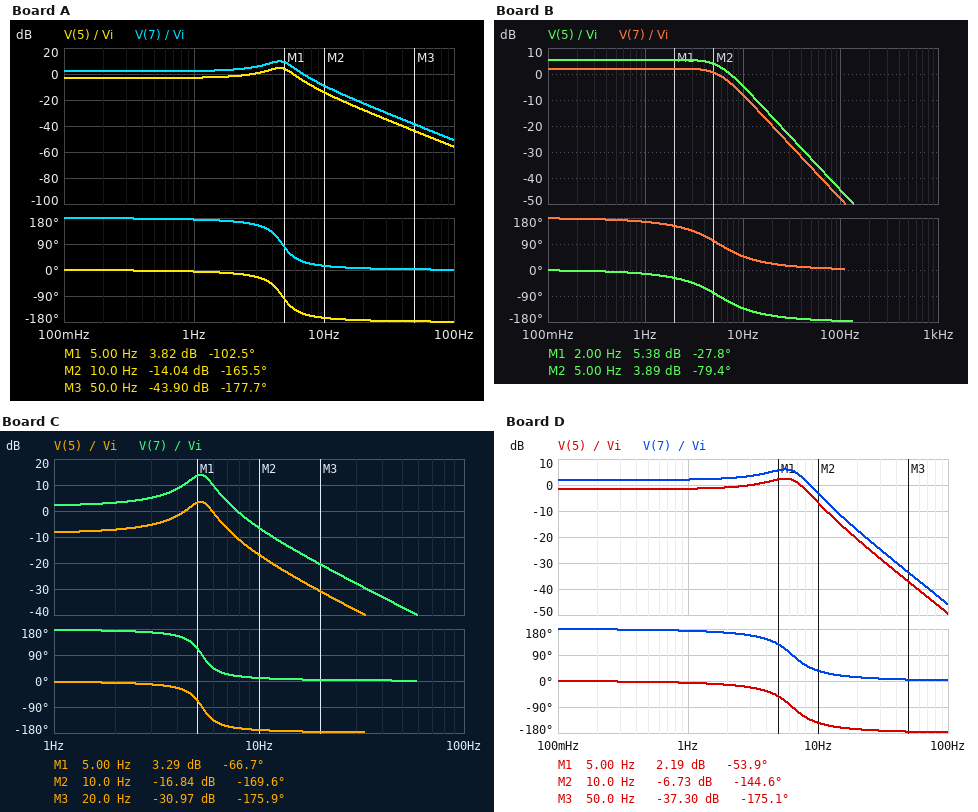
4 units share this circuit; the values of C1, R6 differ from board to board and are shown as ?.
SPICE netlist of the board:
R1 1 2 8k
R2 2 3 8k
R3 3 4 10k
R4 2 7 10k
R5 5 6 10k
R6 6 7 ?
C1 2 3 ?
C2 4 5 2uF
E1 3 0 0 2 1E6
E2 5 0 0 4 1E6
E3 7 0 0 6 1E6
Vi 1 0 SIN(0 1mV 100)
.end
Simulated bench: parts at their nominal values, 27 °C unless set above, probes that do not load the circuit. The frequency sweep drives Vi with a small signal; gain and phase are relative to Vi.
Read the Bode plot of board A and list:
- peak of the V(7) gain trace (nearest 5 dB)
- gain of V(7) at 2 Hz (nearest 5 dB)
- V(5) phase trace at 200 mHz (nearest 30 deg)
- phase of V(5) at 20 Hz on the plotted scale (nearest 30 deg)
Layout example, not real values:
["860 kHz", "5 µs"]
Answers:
["10 dB", "5 dB", "0 deg", "-180 deg"]
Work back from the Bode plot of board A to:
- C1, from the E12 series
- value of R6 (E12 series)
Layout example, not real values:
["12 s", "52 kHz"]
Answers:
["10 µF", "18 kΩ"]
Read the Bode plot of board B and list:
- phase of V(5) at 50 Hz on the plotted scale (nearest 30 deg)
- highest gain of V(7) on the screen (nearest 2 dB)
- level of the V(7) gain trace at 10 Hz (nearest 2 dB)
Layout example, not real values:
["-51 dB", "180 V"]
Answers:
["-180 deg", "2 dB", "-8 dB"]
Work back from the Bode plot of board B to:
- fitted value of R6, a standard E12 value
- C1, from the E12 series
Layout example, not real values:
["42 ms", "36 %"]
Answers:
["6.8 kΩ", "2.7 µF"]
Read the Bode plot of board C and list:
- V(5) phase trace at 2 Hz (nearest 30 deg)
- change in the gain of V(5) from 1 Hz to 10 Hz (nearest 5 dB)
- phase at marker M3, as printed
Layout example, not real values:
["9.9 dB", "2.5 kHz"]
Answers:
["0 deg", "-10 dB", "-175.9 deg"]
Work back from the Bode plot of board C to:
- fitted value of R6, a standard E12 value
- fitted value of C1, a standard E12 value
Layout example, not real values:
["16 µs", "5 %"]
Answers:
["33 kΩ", "15 µF"]
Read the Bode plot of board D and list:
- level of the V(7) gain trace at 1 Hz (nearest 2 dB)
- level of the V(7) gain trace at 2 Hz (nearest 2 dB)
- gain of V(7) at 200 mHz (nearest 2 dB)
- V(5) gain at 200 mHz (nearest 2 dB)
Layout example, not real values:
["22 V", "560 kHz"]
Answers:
["2 dB", "2 dB", "2 dB", "-2 dB"]
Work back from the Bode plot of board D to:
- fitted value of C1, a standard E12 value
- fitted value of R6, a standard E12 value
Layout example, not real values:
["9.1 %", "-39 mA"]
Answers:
["4.7 µF", "15 kΩ"]
